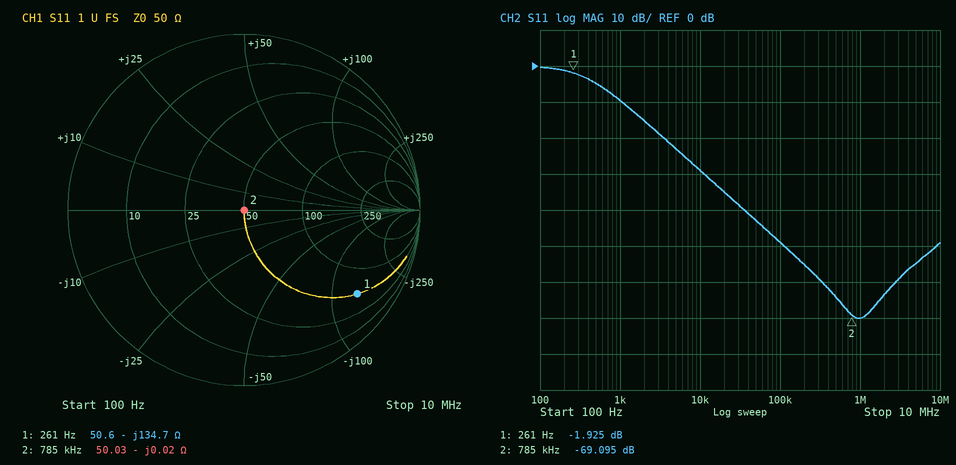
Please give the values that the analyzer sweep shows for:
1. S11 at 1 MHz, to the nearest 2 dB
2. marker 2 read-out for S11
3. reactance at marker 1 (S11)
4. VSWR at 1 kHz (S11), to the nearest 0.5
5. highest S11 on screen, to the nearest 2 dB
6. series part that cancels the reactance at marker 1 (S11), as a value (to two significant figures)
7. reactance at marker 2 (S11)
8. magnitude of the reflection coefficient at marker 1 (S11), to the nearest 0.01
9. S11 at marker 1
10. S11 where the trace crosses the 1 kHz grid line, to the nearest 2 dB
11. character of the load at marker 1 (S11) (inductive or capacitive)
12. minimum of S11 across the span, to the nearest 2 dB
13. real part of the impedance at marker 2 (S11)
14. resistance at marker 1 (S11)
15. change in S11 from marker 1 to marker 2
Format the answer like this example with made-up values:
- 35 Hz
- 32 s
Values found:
- -70 dB
- -69.095 dB
- -134.7 Ω
- 2.0
- 0 dB
- 82 mH
- -0.02 Ω
- 0.80
- -1.925 dB
- -10 dB
- capacitive
- -70 dB
- 50.03 Ω
- 50.6 Ω
- -67.170 dB
